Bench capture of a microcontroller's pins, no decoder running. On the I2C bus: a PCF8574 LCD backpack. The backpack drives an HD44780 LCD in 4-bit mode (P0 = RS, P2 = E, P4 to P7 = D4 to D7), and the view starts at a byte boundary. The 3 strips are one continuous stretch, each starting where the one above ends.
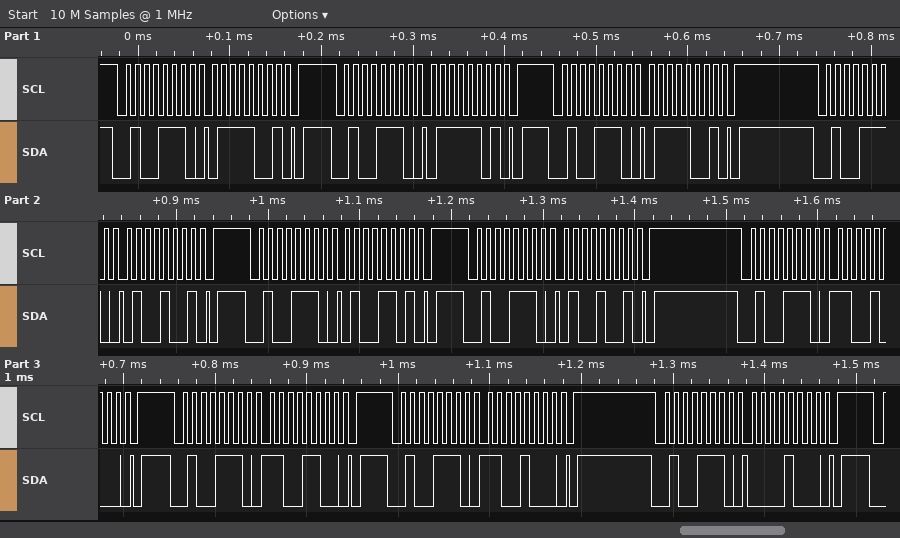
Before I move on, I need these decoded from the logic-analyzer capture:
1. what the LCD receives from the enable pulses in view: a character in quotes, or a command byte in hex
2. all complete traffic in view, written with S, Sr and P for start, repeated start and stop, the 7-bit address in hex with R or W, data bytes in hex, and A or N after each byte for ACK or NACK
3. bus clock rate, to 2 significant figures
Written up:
't'
S 27W A 79 A P S 27W A 7D A P S 27W A 79 A P S 27W A 49 A P S 27W A 4D A P S 27W A 49 A P S 27W A C8 A P S 27W A CC A P S 27W A C8 A P S 27W A 08 A P
100 kHz
